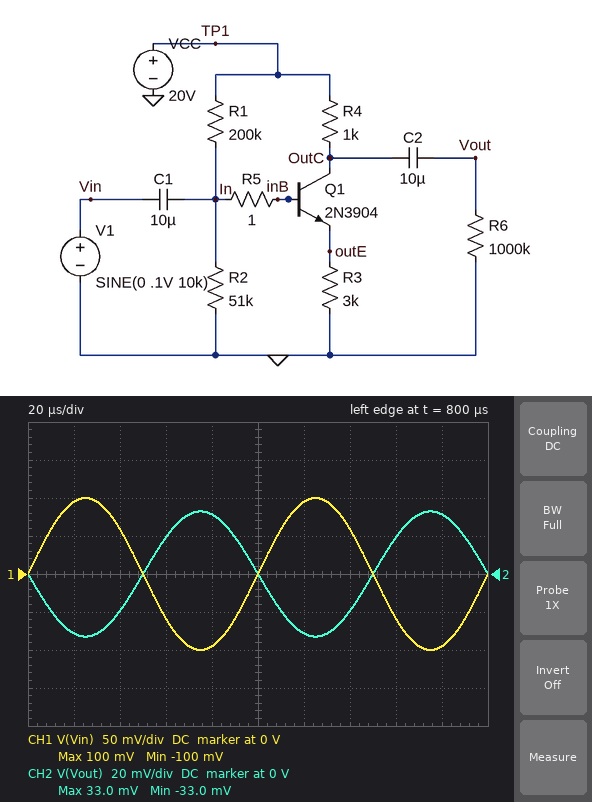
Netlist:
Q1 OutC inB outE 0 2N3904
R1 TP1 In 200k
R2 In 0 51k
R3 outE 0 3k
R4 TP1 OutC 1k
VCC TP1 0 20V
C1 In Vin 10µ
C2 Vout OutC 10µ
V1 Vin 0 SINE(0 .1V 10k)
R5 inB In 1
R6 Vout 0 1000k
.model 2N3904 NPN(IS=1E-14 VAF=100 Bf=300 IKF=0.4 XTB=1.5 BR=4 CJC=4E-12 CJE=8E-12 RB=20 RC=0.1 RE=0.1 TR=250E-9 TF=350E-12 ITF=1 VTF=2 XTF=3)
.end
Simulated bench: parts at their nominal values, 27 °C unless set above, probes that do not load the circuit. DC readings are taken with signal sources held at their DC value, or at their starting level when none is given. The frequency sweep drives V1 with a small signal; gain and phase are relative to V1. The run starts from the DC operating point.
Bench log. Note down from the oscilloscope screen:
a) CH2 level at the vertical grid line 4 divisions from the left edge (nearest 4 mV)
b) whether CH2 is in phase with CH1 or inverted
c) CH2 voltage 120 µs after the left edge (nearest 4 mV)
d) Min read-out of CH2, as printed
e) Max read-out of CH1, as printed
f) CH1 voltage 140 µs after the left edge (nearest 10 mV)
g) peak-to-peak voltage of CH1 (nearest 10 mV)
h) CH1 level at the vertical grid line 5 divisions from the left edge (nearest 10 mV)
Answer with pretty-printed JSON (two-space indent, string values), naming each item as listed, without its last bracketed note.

{
  "CH2 level at the vertical grid line 4 divisions from the left edge": "32 mV",
  "whether CH2 is in phase with CH1 or inverted": "inverted",
  "CH2 voltage 120 µs after the left edge": "-32 mV",
  "Min read-out of CH2, as printed": "-33.0 mV",
  "Max read-out of CH1, as printed": "100 mV",
  "CH1 voltage 140 µs after the left edge": "60 mV",
  "peak-to-peak voltage of CH1": "200 mV",
  "CH1 level at the vertical grid line 5 divisions from the left edge": "0 V"
}
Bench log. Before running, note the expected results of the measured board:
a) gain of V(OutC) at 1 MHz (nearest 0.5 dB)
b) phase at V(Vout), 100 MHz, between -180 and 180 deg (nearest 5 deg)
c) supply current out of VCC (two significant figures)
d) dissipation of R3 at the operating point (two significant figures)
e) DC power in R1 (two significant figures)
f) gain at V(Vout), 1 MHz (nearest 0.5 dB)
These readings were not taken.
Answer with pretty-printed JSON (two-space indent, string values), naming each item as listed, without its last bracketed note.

{
  "gain of V(OutC) at 1 MHz": "-9.5 dB",
  "phase at V(Vout), 100 MHz, between -180 and 180 deg": "60 deg",
  "supply current out of VCC": "1.2 mA",
  "dissipation of R3 at the operating point": "3.6 mW",
  "DC power in R1": "1.3 mW",
  "gain at V(Vout), 1 MHz": "-9.5 dB"
}
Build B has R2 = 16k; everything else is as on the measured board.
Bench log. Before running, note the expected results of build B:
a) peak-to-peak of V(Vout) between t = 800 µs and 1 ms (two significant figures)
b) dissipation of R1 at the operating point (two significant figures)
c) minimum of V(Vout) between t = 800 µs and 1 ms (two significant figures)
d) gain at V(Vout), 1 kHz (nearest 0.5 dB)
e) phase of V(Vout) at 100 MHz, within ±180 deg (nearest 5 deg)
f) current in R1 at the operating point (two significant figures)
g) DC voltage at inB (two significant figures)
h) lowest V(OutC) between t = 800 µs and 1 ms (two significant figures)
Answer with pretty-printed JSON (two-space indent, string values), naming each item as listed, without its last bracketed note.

{
  "peak-to-peak of V(Vout) between t = 800 µs and 1 ms": "64 mV",
  "dissipation of R1 at the operating point": "1.7 mW",
  "minimum of V(Vout) between t = 800 µs and 1 ms": "-32 mV",
  "gain at V(Vout), 1 kHz": "-10.0 dB",
  "phase of V(Vout) at 100 MHz, within ±180 deg": "60 deg",
  "current in R1 at the operating point": "93 µA",
  "DC voltage at inB": "1.5 V",
  "lowest V(OutC) between t = 800 µs and 1 ms": "20 V"
}
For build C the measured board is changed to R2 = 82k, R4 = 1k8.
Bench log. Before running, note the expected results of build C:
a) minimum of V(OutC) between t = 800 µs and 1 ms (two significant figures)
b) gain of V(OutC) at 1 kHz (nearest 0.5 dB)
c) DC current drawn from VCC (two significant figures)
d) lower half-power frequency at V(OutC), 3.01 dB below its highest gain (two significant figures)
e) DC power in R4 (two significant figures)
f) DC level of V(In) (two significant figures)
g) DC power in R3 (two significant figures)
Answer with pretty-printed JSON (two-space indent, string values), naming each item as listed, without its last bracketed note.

{
  "minimum of V(OutC) between t = 800 µs and 1 ms": "17 V",
  "gain of V(OutC) at 1 kHz": "-4.5 dB",
  "DC current drawn from VCC": "1.7 mA",
  "lower half-power frequency at V(OutC), 3.01 dB below its highest gain": "28 MHz",
  "DC power in R4": "4.7 mW",
  "DC level of V(In)": "5.5 V",
  "DC power in R3": "7.9 mW"
}
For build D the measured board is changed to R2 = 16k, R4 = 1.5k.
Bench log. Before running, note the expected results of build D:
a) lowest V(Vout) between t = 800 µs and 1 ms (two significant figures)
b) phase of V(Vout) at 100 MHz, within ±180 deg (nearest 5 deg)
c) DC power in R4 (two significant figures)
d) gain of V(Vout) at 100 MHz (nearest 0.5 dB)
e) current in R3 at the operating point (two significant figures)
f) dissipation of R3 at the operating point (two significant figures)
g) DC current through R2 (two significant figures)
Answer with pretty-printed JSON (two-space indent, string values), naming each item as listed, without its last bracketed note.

{
  "lowest V(Vout) between t = 800 µs and 1 ms": "-48 mV",
  "phase of V(Vout) at 100 MHz, within ±180 deg": "45 deg",
  "DC power in R4": "120 µW",
  "gain of V(Vout) at 100 MHz": "-0.5 dB",
  "current in R3 at the operating point": "280 µA",
  "dissipation of R3 at the operating point": "240 µW",
  "DC current through R2": "92 µA"
}
